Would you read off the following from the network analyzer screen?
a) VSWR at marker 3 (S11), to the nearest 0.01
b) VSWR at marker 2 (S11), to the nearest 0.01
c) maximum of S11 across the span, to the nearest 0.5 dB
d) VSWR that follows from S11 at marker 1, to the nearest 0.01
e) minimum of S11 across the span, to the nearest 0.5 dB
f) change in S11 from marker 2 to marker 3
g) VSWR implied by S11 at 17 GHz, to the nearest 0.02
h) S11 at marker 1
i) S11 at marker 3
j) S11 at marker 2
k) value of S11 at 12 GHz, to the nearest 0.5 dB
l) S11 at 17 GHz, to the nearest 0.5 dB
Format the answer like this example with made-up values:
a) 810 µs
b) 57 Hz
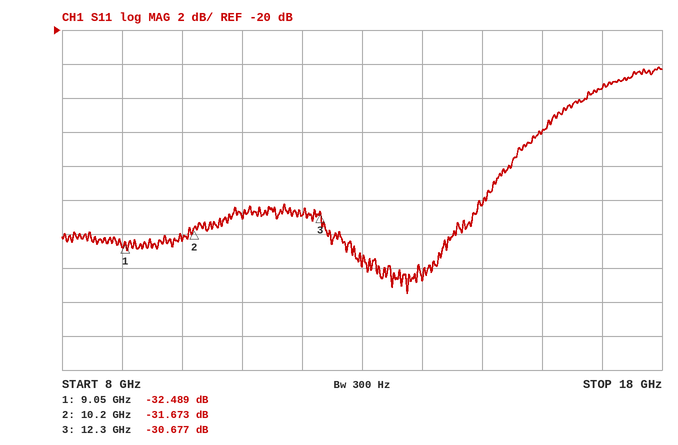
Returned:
a) 1.06
b) 1.05
c) -22.0 dB
d) 1.05
e) -35.5 dB
f) 0.996 dB
g) 1.14
h) -32.489 dB
i) -30.677 dB
j) -31.673 dB
k) -31.0 dB
l) -23.5 dB
